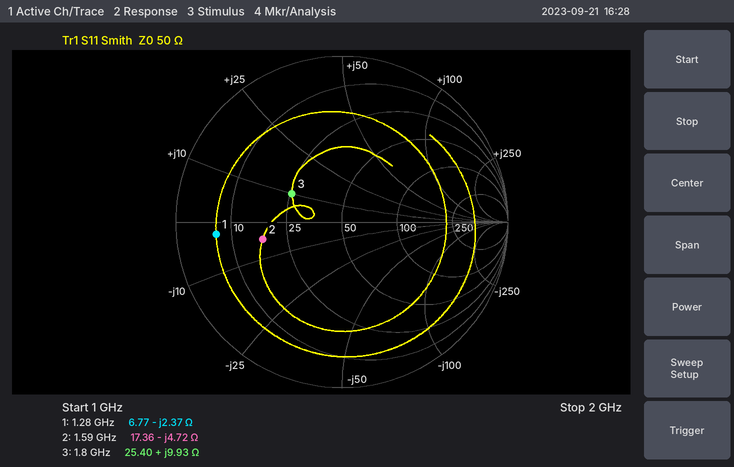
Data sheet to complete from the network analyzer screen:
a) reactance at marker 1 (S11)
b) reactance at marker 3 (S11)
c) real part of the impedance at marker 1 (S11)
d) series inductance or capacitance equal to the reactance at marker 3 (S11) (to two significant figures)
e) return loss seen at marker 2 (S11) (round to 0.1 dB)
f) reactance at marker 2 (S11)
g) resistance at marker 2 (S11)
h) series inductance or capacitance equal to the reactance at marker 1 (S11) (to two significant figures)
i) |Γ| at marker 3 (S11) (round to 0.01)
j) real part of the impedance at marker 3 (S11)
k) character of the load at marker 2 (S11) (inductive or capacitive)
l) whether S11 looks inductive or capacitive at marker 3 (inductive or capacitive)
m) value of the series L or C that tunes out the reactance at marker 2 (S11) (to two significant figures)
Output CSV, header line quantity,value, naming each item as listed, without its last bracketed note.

quantity,value
reactance at marker 1,-2.37 Ω
reactance at marker 3,+9.93 Ω
real part of the impedance at marker 1,6.77 Ω
series inductance or capacitance equal to the reactance at marker 3 (S11),880 pH
return loss seen at marker 2 (S11),6.2 dB
reactance at marker 2,-4.72 Ω
resistance at marker 2,17.36 Ω
series inductance or capacitance equal to the reactance at marker 1 (S11),52 pF
|Γ| at marker 3 (S11),0.35
real part of the impedance at marker 3,25.40 Ω
character of the load at marker 2 (S11),capacitive
whether S11 looks inductive or capacitive at marker 3,inductive
value of the series L or C that tunes out the reactance at marker 2 (S11),470 pH
